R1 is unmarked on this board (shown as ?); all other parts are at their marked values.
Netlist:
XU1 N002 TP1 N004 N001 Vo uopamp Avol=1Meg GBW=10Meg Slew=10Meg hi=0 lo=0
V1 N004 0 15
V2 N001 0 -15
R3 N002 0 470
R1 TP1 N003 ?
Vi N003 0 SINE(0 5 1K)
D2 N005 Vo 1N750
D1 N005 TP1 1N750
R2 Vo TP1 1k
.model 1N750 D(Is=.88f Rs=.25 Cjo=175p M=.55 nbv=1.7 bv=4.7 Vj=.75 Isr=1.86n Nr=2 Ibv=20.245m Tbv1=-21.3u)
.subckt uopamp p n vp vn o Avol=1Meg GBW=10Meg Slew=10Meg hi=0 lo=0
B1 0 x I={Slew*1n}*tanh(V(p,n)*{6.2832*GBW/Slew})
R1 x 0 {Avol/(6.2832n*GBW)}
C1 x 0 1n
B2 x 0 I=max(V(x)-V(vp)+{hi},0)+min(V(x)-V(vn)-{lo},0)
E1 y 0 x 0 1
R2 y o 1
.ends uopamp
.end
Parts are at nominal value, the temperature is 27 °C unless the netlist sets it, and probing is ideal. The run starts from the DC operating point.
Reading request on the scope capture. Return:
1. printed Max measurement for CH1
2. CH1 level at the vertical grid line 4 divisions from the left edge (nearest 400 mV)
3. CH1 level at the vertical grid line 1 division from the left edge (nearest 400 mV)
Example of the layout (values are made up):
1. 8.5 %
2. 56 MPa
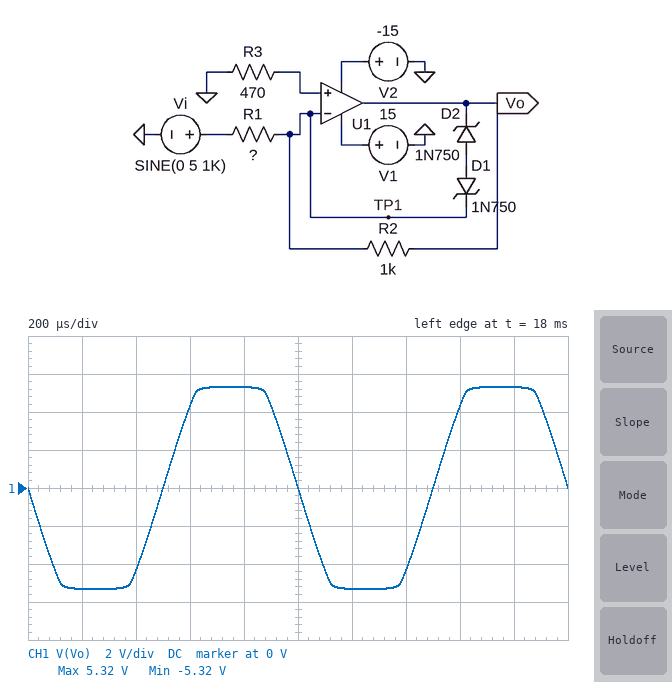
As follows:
1. 5.32 V
2. 5.2 V
3. -5.2 V
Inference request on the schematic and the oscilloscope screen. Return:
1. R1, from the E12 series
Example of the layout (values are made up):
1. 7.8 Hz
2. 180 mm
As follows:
1. 680 Ω
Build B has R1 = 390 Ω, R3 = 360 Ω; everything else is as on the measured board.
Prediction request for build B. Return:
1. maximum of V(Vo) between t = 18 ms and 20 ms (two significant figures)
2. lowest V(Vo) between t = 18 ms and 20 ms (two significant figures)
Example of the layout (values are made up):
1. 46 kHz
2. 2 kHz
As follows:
1. 5.4 V
2. -5.4 V
